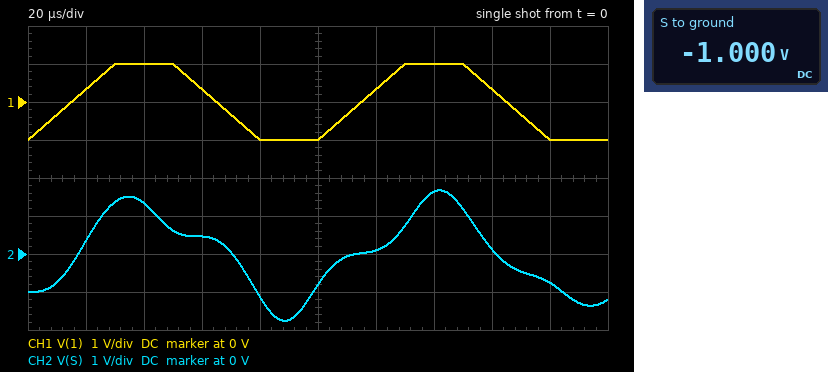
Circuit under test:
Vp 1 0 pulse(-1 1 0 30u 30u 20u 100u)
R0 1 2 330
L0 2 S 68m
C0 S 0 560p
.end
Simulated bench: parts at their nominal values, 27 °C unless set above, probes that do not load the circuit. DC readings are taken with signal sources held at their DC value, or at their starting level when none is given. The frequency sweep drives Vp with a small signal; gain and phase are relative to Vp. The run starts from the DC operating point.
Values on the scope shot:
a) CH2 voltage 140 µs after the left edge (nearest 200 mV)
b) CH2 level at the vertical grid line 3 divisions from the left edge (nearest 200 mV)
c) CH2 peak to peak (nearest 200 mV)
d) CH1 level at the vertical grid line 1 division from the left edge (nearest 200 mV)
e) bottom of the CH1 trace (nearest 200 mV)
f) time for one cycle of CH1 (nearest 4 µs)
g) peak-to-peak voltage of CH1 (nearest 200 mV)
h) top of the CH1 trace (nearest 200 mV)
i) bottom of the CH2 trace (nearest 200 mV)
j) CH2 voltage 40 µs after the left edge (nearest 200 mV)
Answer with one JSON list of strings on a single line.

["1.6 V", "400 mV", "3.4 V", "400 mV", "-1.0 V", "100 µs", "2.0 V", "1.0 V", "-1.8 V", "1.4 V"]
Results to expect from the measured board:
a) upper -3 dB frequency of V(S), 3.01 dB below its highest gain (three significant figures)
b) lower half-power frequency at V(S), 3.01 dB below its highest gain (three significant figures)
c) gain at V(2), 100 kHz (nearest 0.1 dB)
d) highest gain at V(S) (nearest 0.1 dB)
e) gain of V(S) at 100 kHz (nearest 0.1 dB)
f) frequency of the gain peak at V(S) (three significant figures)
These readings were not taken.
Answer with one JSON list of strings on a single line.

["26.2 kHz", "25.4 kHz", "0 dB", "30.5 dB", "-22.9 dB", "25.8 kHz"]
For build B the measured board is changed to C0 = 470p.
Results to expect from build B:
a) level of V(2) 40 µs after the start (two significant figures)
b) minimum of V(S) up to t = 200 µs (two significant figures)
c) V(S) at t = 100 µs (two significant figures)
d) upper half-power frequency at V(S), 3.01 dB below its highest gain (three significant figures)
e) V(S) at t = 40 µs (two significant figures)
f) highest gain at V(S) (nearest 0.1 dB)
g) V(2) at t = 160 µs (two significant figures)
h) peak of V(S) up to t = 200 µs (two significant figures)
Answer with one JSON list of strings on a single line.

["1.0 V", "-1.9 V", "-470 mV", "28.5 kHz", "1.1 V", "31.2 dB", "330 mV", "1.8 V"]
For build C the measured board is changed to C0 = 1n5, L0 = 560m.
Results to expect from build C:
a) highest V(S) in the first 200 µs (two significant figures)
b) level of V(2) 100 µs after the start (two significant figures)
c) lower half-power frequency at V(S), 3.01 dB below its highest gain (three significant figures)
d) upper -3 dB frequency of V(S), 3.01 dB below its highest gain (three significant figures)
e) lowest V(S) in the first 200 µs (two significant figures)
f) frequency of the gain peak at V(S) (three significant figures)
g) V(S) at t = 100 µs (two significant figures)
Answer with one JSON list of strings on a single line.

["1.9 V", "-980 mV", "5.44 kHz", "5.54 kHz", "-1.4 V", "5.49 kHz", "1.5 V"]
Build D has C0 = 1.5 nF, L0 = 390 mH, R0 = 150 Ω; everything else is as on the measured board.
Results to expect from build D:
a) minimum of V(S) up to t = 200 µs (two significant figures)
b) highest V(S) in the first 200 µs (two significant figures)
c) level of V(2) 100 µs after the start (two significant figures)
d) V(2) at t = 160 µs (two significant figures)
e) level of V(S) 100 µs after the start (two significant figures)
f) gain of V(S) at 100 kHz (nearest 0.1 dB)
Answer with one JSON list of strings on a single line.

["-2.6 V", "2.2 V", "-980 mV", "310 mV", "960 mV", "-47.2 dB"]
